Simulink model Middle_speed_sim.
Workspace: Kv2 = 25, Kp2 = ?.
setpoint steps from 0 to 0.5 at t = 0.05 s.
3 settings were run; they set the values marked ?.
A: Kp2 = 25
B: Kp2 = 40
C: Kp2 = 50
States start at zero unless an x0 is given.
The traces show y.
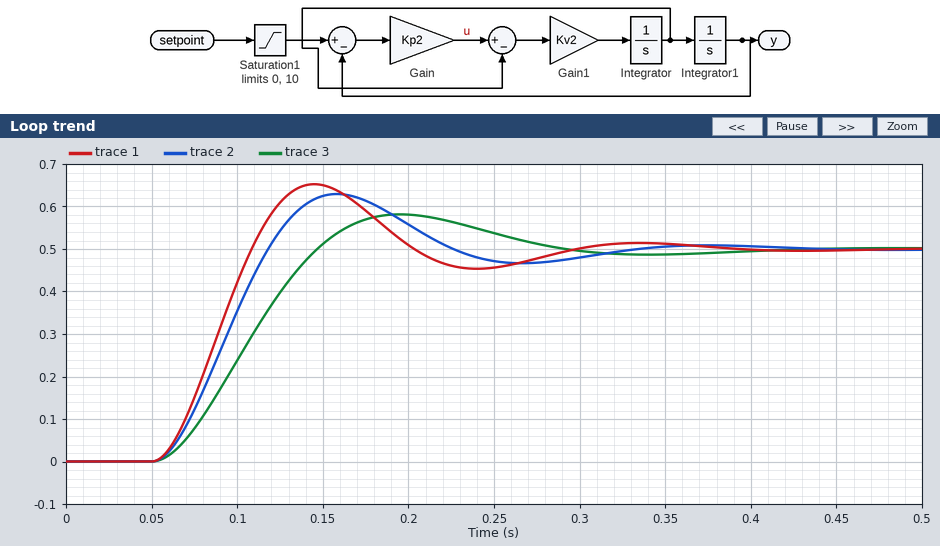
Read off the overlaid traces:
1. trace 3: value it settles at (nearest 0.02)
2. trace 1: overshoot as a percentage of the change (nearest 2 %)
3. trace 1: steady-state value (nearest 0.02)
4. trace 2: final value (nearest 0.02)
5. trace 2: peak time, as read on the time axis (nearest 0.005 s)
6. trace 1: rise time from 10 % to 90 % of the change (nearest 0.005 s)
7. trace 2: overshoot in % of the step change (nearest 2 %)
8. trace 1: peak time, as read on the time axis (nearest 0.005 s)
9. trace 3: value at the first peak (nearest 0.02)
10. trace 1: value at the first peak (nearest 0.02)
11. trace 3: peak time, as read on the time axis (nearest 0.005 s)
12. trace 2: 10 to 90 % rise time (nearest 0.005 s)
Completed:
0.50
30 %
0.50
0.50
0.160 s
0.040 s
26 %
0.145 s
0.58
0.66
0.195 s
0.045 s
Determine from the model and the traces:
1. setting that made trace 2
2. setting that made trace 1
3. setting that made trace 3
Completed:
B
C
A
